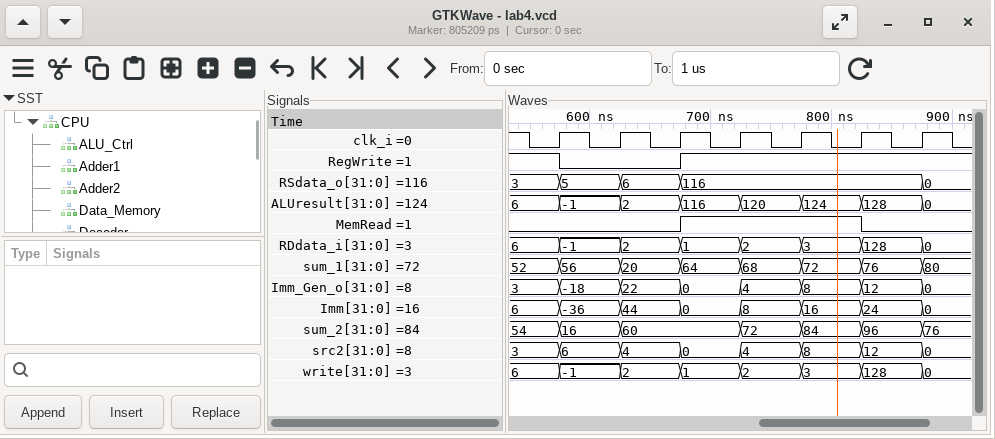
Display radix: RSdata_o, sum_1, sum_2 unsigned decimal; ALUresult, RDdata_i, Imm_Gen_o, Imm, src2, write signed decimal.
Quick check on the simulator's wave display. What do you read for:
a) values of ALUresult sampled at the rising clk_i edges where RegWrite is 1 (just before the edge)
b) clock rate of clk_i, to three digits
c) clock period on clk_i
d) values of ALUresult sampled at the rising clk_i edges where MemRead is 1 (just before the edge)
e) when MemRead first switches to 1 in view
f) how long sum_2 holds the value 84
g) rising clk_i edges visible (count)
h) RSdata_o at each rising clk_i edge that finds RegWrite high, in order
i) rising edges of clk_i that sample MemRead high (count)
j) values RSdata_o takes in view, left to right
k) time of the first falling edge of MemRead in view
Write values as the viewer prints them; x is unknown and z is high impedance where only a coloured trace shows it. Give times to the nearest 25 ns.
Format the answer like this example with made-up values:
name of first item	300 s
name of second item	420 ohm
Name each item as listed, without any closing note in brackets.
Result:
values of ALUresult sampled at the rising clk_i edges where RegWrite is 1	6, 116, 120, 124, 128
clock rate of clk_i, to three digits	20.0 MHz
clock period on clk_i	50 ns
values of ALUresult sampled at the rising clk_i edges where MemRead is 1	116, 120, 124
when MemRead first switches to 1 in view	675 ns
how long sum_2 holds the value 84	50 ns
rising clk_i edges visible	7
RSdata_o at each rising clk_i edge that finds RegWrite high, in order	3, 116, 116, 116, 116
rising edges of clk_i that sample MemRead high	3
values RSdata_o takes in view, left to right	3, 5, 6, 116, 0
time of the first falling edge of MemRead in view	825 ns
